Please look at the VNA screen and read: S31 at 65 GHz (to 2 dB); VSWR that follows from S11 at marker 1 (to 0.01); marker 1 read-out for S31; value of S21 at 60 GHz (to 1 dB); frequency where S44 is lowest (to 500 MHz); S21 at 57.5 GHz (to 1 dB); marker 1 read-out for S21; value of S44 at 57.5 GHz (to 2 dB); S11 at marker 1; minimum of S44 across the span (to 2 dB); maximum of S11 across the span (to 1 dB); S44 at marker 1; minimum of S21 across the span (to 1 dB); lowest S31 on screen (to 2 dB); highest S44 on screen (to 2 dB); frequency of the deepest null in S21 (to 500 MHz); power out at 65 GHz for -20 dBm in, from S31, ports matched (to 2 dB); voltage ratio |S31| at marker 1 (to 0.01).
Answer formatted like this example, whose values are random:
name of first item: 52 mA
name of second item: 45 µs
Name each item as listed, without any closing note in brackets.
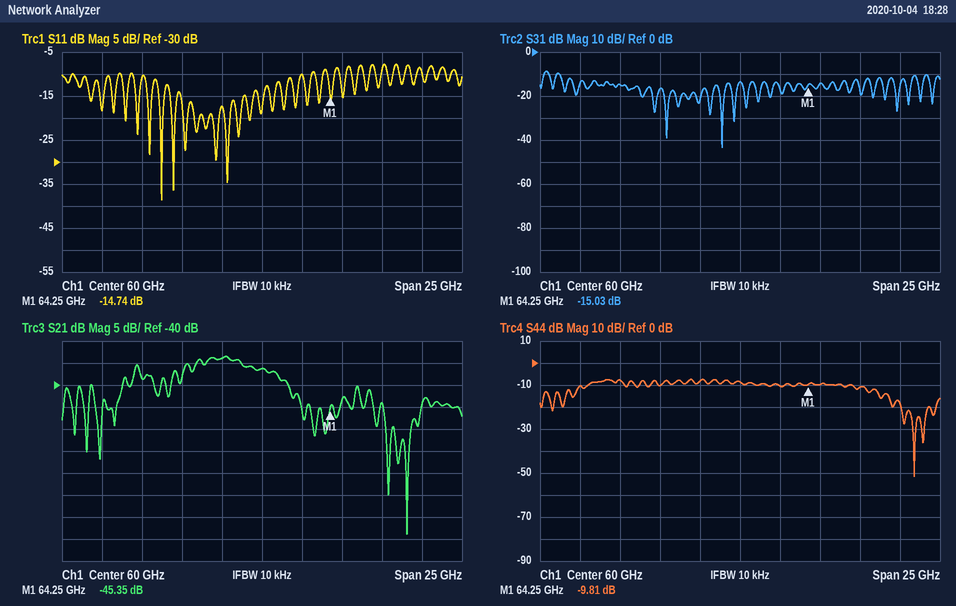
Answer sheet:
S31 at 65 GHz: -14 dB
VSWR that follows from S11 at marker 1: 1.45
marker 1 read-out for S31: -15.03 dB
value of S21 at 60 GHz: -36 dB
frequency where S44 is lowest: 71.0 GHz
S21 at 57.5 GHz: -34 dB
marker 1 read-out for S21: -45.35 dB
value of S44 at 57.5 GHz: -8 dB
S11 at marker 1: -14.74 dB
minimum of S44 across the span: -52 dB
maximum of S11 across the span: -8 dB
S44 at marker 1: -9.81 dB
minimum of S21 across the span: -74 dB
lowest S31 on screen: -44 dB
highest S44 on screen: -8 dB
frequency of the deepest null in S21: 69.0 GHz
power out at 65 GHz for -20 dBm in, from S31, ports matched: -34 dBm
voltage ratio |S31| at marker 1: 0.18
